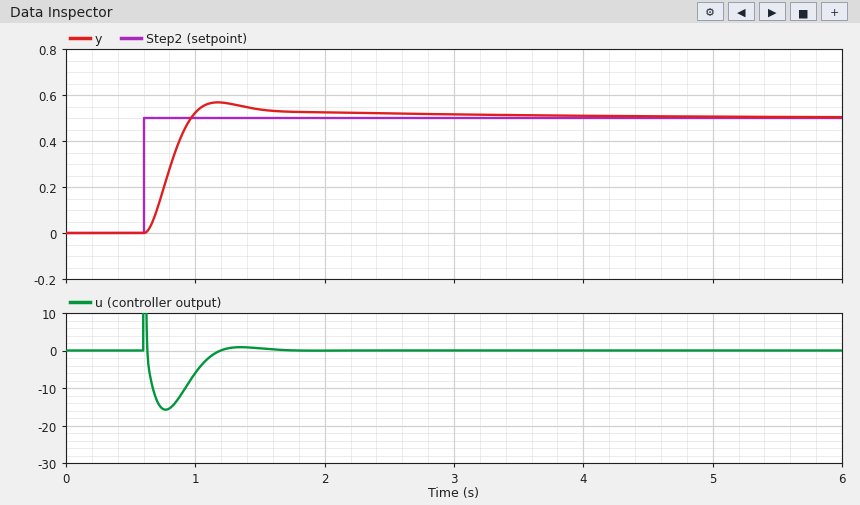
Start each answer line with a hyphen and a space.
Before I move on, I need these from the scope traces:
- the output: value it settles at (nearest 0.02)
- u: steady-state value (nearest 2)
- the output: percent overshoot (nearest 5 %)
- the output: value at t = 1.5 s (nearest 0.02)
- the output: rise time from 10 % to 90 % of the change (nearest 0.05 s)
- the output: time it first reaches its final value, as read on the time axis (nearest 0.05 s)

- 0.50
- 0
- 15 %
- 0.54
- 0.25 s
- 0.95 s
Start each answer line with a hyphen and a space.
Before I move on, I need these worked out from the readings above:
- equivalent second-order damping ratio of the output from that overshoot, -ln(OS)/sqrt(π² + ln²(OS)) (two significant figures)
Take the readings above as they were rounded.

- 0.52
